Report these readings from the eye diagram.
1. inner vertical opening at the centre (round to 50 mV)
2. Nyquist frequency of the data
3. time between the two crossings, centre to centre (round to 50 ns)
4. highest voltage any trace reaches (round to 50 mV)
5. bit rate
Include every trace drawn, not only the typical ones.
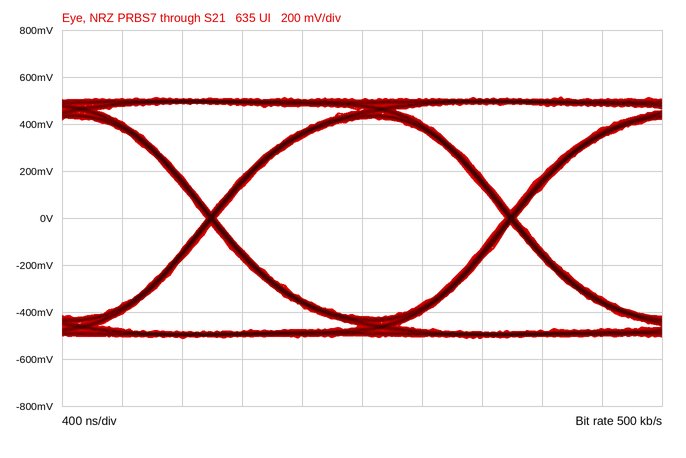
850 mV
250 kHz
2.00 µs
500 mV
500 kb/s
